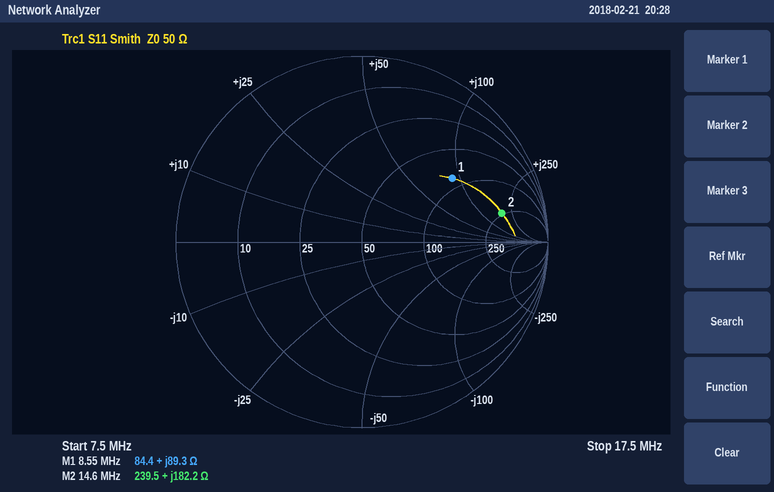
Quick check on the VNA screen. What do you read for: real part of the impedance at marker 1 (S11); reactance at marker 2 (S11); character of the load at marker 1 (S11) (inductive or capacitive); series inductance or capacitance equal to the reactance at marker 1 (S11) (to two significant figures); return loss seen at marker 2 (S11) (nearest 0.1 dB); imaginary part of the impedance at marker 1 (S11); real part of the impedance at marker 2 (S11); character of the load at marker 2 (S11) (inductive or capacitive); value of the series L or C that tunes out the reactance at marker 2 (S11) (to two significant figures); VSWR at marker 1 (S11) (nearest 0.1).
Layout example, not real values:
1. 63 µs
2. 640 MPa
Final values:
1. 84.4 Ω
2. +182.2 Ω
3. inductive
4. 1.7 µH
5. 2.3 dB
6. +89.3 Ω
7. 239.5 Ω
8. inductive
9. 60 pF
10. 3.9
